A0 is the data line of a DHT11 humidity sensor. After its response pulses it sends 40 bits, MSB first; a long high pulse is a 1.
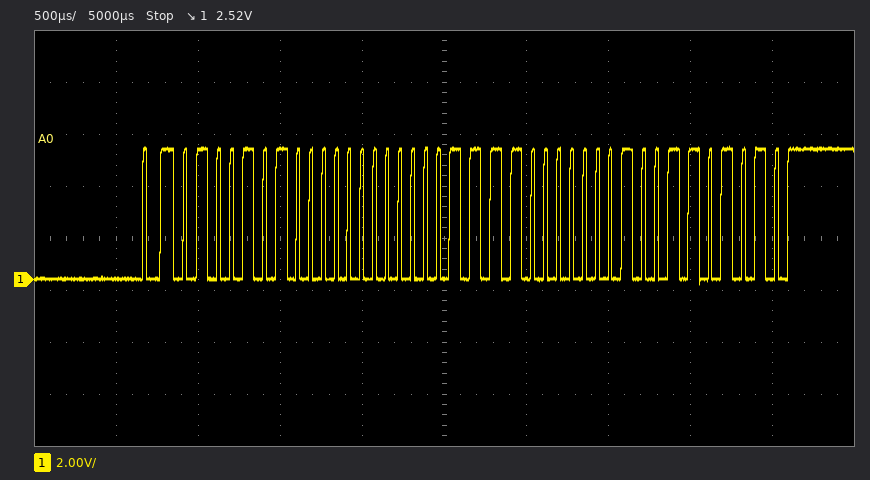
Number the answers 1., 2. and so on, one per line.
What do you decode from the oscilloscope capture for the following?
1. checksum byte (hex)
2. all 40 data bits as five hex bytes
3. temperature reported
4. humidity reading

1. 0x6A
2. 4A 00 1E 02 6A
3. 30.2 °C
4. 74 %
